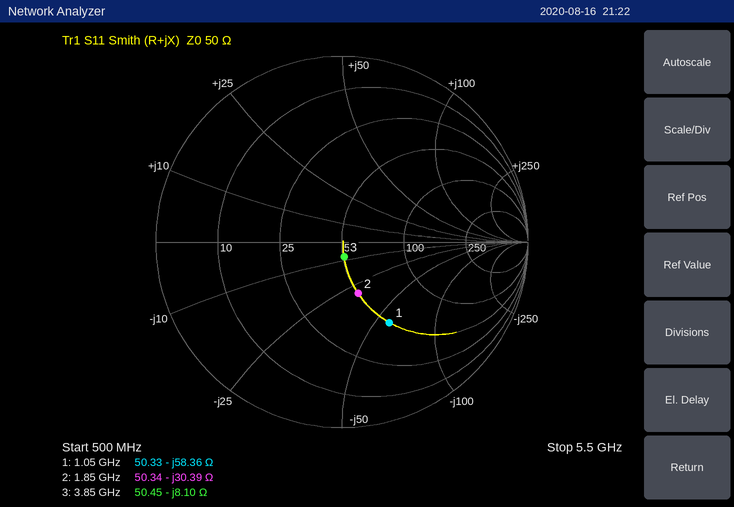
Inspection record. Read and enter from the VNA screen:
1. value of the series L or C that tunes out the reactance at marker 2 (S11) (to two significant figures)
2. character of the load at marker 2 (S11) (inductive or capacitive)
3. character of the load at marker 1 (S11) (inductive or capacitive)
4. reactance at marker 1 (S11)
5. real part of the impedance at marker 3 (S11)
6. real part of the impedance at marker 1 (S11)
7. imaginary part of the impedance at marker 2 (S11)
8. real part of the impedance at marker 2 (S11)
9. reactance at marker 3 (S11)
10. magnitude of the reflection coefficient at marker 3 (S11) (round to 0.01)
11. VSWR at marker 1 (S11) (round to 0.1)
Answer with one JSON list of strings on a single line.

["2.6 nH", "capacitive", "capacitive", "-58.36 Ω", "50.45 Ω", "50.33 Ω", "-30.39 Ω", "50.34 Ω", "-8.10 Ω", "0.08", "3.0"]
